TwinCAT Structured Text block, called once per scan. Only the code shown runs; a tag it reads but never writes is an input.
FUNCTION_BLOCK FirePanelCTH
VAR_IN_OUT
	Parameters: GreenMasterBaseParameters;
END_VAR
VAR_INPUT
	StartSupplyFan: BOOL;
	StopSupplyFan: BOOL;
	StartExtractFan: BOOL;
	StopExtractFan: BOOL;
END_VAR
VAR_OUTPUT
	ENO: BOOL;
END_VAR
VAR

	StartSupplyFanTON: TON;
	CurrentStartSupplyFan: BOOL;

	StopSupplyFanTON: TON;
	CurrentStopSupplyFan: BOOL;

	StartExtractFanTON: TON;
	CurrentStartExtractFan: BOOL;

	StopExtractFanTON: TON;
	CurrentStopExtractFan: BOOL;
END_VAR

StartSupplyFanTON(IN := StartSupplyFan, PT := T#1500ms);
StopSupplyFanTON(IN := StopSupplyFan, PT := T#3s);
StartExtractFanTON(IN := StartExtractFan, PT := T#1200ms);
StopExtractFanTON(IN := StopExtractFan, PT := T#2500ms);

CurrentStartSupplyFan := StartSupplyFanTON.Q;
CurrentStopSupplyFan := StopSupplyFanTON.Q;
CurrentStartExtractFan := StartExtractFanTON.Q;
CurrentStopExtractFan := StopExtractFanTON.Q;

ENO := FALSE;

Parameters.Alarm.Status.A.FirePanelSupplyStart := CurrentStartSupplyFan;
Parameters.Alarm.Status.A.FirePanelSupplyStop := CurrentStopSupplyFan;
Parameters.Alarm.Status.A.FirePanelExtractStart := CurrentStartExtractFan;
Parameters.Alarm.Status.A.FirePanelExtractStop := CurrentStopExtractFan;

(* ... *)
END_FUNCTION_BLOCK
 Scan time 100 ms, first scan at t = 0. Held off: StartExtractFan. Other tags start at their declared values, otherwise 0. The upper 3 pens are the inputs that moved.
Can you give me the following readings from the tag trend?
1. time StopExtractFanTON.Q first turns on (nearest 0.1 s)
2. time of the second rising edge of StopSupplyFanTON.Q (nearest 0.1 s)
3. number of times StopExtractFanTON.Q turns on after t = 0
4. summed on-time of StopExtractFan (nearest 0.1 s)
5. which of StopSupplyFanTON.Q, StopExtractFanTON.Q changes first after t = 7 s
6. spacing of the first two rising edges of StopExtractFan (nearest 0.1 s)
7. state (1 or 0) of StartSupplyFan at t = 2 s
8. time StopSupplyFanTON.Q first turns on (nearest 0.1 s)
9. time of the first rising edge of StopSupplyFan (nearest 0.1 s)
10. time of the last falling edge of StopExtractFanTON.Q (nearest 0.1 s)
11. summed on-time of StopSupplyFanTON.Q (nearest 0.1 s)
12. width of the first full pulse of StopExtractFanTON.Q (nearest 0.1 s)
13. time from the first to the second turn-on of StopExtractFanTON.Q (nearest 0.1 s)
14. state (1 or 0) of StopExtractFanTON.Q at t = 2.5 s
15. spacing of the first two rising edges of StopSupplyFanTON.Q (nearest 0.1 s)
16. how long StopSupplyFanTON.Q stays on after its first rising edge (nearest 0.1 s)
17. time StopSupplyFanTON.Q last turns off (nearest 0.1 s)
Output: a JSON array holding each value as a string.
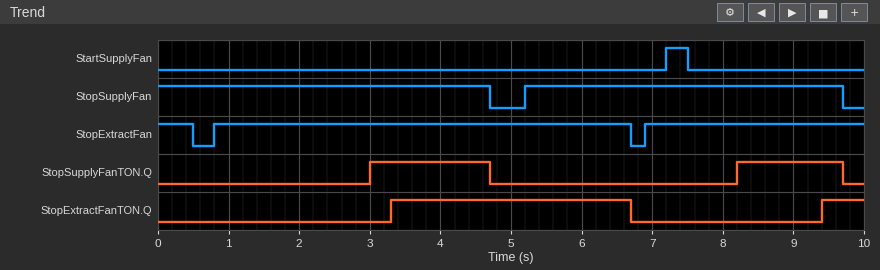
["3.3 s", "8.2 s", "2", "9.5 s", "StopSupplyFanTON.Q", "6.1 s", "0", "3.0 s", "5.2 s", "6.7 s", "3.2 s", "3.4 s", "6.1 s", "0", "5.2 s", "1.7 s", "9.7 s"]
